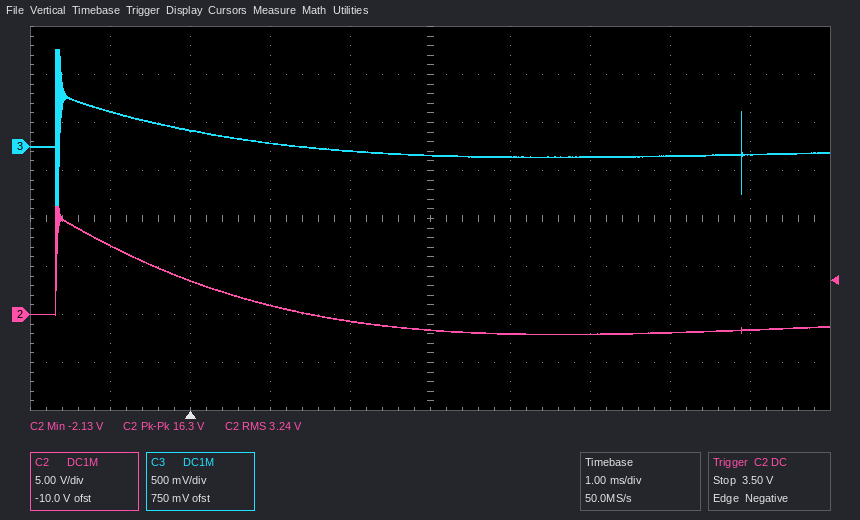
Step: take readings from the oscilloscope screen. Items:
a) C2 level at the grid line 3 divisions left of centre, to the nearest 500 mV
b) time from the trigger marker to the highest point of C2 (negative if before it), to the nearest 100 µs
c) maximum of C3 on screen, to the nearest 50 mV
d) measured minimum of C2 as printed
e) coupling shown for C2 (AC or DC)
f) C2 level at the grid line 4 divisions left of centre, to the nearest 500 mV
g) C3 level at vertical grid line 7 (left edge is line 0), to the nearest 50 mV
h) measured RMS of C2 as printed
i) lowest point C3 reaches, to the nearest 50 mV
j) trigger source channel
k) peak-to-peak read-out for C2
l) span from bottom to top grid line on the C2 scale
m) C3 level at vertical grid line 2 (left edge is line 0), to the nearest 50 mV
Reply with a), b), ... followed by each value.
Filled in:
a) 3.5 V
b) -1.7 ms
c) 1.00 V
d) -2.13 V
e) DC
f) 7.0 V
g) -100 mV
h) 3.24 V
i) -600 mV
j) C2
k) 16.3 V
l) 40 V
m) 150 mV
